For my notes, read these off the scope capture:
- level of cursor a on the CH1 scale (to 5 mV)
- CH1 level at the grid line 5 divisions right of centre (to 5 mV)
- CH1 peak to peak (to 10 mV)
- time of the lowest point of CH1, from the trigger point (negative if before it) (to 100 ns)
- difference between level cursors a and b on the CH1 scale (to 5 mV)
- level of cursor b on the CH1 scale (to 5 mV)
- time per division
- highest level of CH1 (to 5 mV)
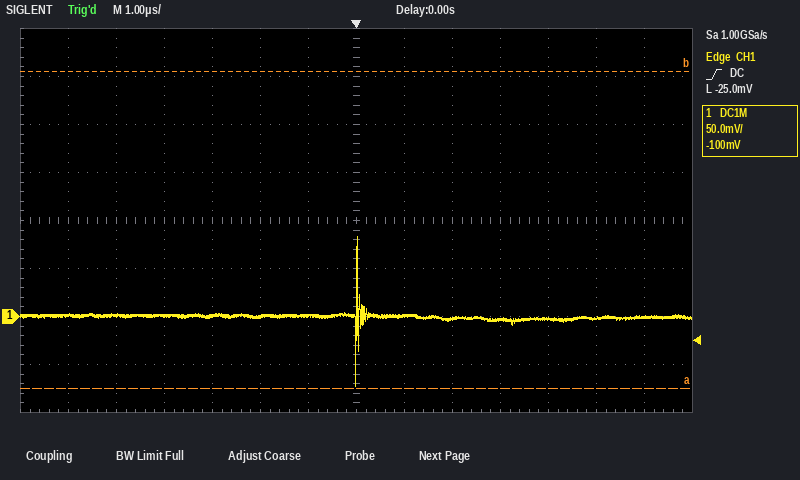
-75 mV
0 mV
160 mV
0.0 µs
330 mV
255 mV
1 µs
85 mV
